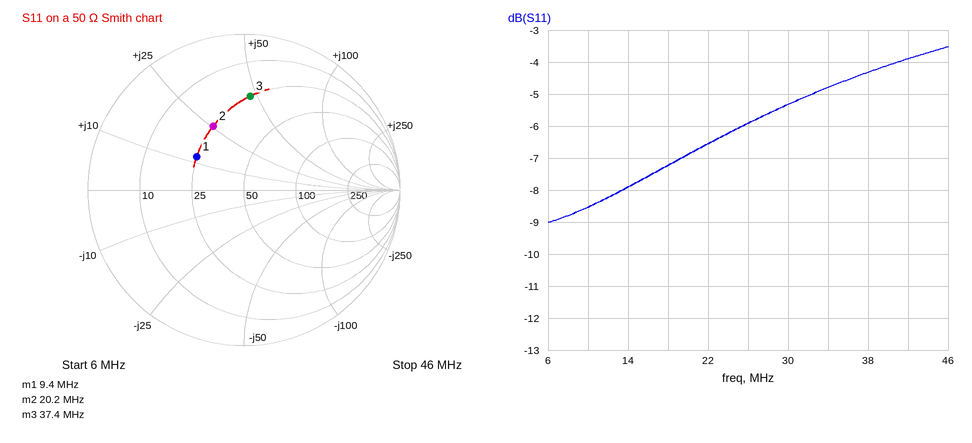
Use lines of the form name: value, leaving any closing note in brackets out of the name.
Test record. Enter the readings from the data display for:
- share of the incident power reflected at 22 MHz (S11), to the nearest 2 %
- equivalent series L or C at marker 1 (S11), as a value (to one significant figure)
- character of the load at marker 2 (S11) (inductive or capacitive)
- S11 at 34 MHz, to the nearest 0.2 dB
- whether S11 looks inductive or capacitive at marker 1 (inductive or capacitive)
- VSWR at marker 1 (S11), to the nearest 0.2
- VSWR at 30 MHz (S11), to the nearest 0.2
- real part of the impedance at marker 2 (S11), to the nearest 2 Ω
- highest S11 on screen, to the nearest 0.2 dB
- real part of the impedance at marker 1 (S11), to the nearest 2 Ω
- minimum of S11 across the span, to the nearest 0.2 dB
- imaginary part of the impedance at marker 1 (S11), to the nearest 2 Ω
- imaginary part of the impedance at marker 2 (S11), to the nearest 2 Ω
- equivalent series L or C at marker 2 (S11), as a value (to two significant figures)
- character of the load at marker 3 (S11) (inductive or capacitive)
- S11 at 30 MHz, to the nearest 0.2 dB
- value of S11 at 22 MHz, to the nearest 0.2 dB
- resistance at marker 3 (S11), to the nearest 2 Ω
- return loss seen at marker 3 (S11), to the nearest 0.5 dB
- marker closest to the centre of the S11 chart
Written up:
share of the incident power reflected at 22 MHz (S11), to the nearest 2 %: 22 %
equivalent series L or C at marker 1 (S11), as a value: 200 nH
character of the load at marker 2 (S11): inductive
S11 at 34 MHz, to the nearest 0.2 dB: -4.8 dB
whether S11 looks inductive or capacitive at marker 1: inductive
VSWR at marker 1 (S11), to the nearest 0.2: 2.2
VSWR at 30 MHz (S11), to the nearest 0.2: 3.4
real part of the impedance at marker 2 (S11), to the nearest 2 Ω: 24 Ω
highest S11 on screen, to the nearest 0.2 dB: -3.6 dB
real part of the impedance at marker 1 (S11), to the nearest 2 Ω: 24 Ω
minimum of S11 across the span, to the nearest 0.2 dB: -9.0 dB
imaginary part of the impedance at marker 1 (S11), to the nearest 2 Ω: +12 Ω
imaginary part of the impedance at marker 2 (S11), to the nearest 2 Ω: +26 Ω
equivalent series L or C at marker 2 (S11), as a value: 200 nH
character of the load at marker 3 (S11): inductive
S11 at 30 MHz, to the nearest 0.2 dB: -5.4 dB
value of S11 at 22 MHz, to the nearest 0.2 dB: -6.6 dB
resistance at marker 3 (S11), to the nearest 2 Ω: 24 Ω
return loss seen at marker 3 (S11), to the nearest 0.5 dB: 4.5 dB
marker closest to the centre of the S11 chart: marker 1
